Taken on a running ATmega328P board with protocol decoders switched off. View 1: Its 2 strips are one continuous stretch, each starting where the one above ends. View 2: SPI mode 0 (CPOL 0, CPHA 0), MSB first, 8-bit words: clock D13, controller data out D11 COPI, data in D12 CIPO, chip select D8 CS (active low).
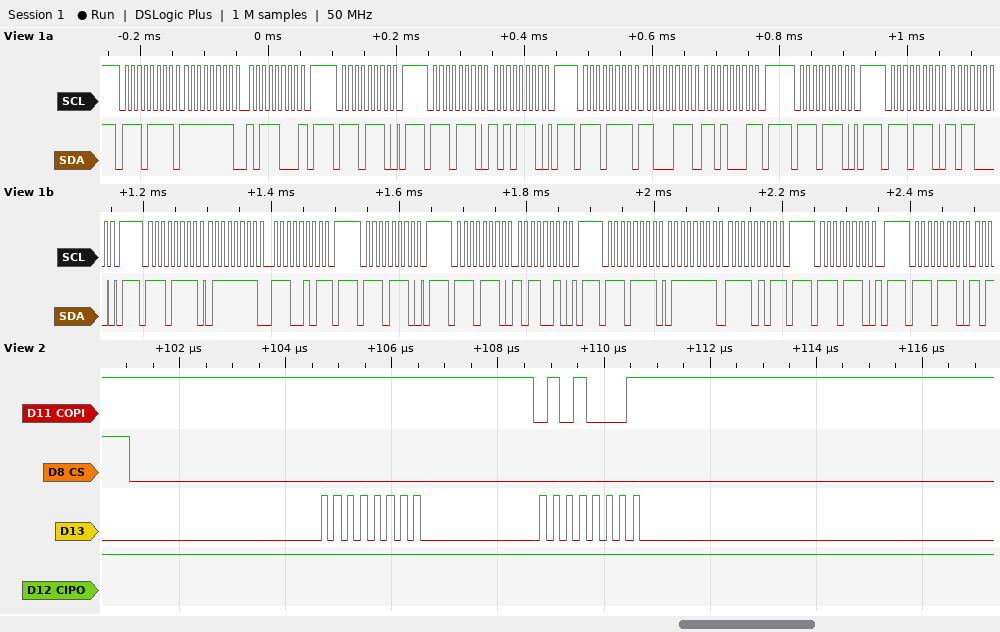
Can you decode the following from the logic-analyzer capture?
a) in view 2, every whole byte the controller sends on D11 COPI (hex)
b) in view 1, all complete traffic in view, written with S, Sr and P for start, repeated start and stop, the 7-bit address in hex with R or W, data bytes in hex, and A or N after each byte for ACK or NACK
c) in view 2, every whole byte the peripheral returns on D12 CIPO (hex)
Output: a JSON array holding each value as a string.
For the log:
["FF 51", "S 77R A FF A B8 N P S 77W A P S 77W A AE A P S 77R A C7 A D1 N P S 77W A P S 77W A B0 A P S 77R A 7F A E5 N P S 77W A P S 77W A B2 A P S 77R A 7F A F5 N P S 77W A P S 77W A", "FF FF"]
